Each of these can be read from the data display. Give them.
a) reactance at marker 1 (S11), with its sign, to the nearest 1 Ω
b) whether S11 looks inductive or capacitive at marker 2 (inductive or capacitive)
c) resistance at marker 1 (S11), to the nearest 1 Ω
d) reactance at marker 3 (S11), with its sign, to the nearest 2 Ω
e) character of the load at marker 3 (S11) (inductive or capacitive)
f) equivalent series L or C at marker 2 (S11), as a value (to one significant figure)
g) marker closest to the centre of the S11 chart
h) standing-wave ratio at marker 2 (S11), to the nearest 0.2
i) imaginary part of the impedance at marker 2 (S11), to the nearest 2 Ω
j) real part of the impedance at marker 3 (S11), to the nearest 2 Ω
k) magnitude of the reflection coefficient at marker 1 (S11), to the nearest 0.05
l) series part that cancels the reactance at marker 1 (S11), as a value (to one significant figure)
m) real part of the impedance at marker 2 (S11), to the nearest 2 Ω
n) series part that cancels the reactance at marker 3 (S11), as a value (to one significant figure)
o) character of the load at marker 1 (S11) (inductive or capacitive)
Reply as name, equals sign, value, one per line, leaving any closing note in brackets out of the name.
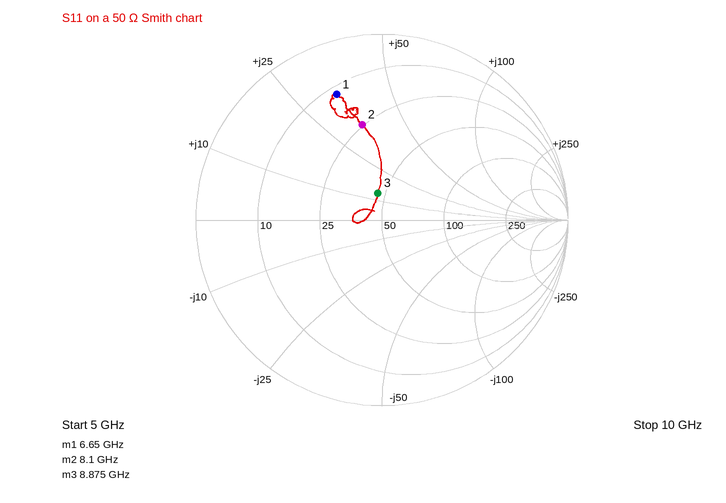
reactance at marker 1 (S11), with its sign, to the nearest 1 Ω = +34 Ω
whether S11 looks inductive or capacitive at marker 2 = inductive
resistance at marker 1 (S11), to the nearest 1 Ω = 12 Ω
reactance at marker 3 (S11), with its sign, to the nearest 2 Ω = +14 Ω
character of the load at marker 3 (S11) = inductive
equivalent series L or C at marker 2 (S11), as a value = 700 pH
marker closest to the centre of the S11 chart = marker 3
standing-wave ratio at marker 2 (S11), to the nearest 0.2 = 3.2
imaginary part of the impedance at marker 2 (S11), to the nearest 2 Ω = +34 Ω
real part of the impedance at marker 3 (S11), to the nearest 2 Ω = 46 Ω
magnitude of the reflection coefficient at marker 1 (S11), to the nearest 0.05 = 0.70
series part that cancels the reactance at marker 1 (S11), as a value = 700 fF
real part of the impedance at marker 2 (S11), to the nearest 2 Ω = 24 Ω
series part that cancels the reactance at marker 3 (S11), as a value = 1 pF
character of the load at marker 1 (S11) = inductive
